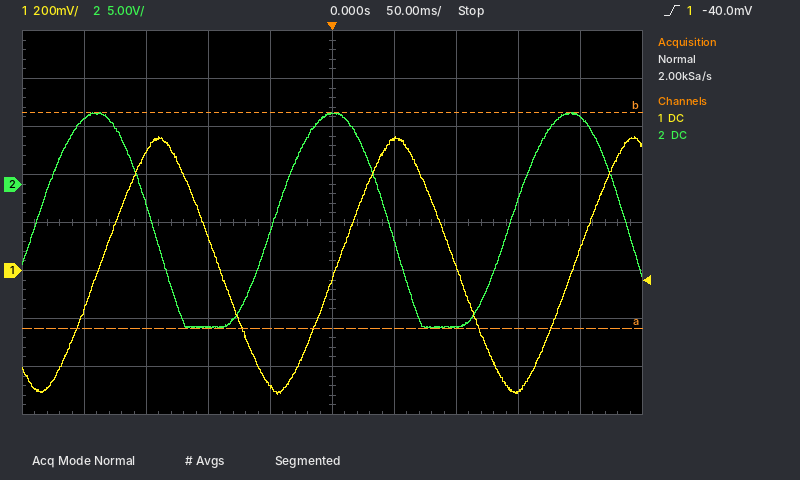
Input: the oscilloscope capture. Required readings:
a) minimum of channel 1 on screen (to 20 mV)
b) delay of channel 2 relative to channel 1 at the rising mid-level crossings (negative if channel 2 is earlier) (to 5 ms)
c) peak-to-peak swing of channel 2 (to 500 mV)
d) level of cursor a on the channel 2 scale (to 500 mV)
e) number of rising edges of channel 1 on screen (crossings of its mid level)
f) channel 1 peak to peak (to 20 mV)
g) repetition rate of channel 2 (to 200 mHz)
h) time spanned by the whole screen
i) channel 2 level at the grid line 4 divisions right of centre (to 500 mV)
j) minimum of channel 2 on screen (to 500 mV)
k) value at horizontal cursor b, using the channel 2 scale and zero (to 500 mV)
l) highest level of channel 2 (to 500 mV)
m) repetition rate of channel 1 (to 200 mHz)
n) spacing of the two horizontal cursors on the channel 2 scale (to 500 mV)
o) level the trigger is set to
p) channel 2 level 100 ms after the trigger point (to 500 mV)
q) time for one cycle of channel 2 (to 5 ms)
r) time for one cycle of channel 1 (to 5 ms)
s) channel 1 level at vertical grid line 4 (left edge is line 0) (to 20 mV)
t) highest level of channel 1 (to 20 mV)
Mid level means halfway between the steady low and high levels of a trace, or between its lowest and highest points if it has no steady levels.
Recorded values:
-520 mV
-50 ms
22.5 V
-15.0 V
3
1.08 V
5.2 Hz
500 ms
7.0 V
-15.0 V
7.5 V
7.5 V
5.2 Hz
22.5 V
-40.0 mV
-15.0 V
190 ms
190 ms
-480 mV
560 mV
